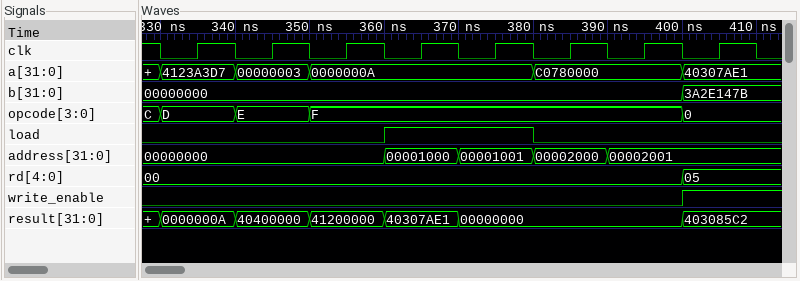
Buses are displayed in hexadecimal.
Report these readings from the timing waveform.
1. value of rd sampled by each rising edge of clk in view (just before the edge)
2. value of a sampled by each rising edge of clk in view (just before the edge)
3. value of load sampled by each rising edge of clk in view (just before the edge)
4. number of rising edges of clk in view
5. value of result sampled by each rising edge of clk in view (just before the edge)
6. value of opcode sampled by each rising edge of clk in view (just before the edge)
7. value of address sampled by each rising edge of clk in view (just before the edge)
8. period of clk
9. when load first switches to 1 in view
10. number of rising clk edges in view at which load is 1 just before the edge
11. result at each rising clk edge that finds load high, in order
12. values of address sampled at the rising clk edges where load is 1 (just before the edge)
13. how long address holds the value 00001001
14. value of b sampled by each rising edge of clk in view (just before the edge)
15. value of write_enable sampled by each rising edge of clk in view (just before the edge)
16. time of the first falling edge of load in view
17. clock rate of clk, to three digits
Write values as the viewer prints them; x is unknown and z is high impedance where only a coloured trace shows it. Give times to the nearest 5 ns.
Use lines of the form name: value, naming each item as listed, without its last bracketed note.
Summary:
value of rd sampled by each rising edge of clk in view: 00, 00, 00, 00, 00, 00, 00, 05
value of a sampled by each rising edge of clk in view: 4123A3D7, 00000003, 0000000A, 0000000A, 0000000A, C0780000, C0780000, 40307AE1
value of load sampled by each rising edge of clk in view: 0 0 0 1 1 0 0 0
number of rising edges of clk in view: 8
value of result sampled by each rising edge of clk in view: 0000000A, 40400000, 41200000, 40307AE1, 00000000, 00000000, 00000000, 403085C2
value of opcode sampled by each rising edge of clk in view: D, E, F, F, F, F, F, 0
value of address sampled by each rising edge of clk in view: 00000000, 00000000, 00000000, 00001000, 00001001, 00002000, 00002001, 00002001
period of clk: 10 ns
when load first switches to 1 in view: 360 ns
number of rising clk edges in view at which load is 1 just before the edge: 2
result at each rising clk edge that finds load high, in order: 40307AE1, 00000000
values of address sampled at the rising clk edges where load is 1: 00001000, 00001001
how long address holds the value 00001001: 10 ns
value of b sampled by each rising edge of clk in view: 00000000, 00000000, 00000000, 00000000, 00000000, 00000000, 00000000, 3A2E147B
value of write_enable sampled by each rising edge of clk in view: 0 0 0 0 0 0 0 1
time of the first falling edge of load in view: 380 ns
clock rate of clk, to three digits: 100 MHz
